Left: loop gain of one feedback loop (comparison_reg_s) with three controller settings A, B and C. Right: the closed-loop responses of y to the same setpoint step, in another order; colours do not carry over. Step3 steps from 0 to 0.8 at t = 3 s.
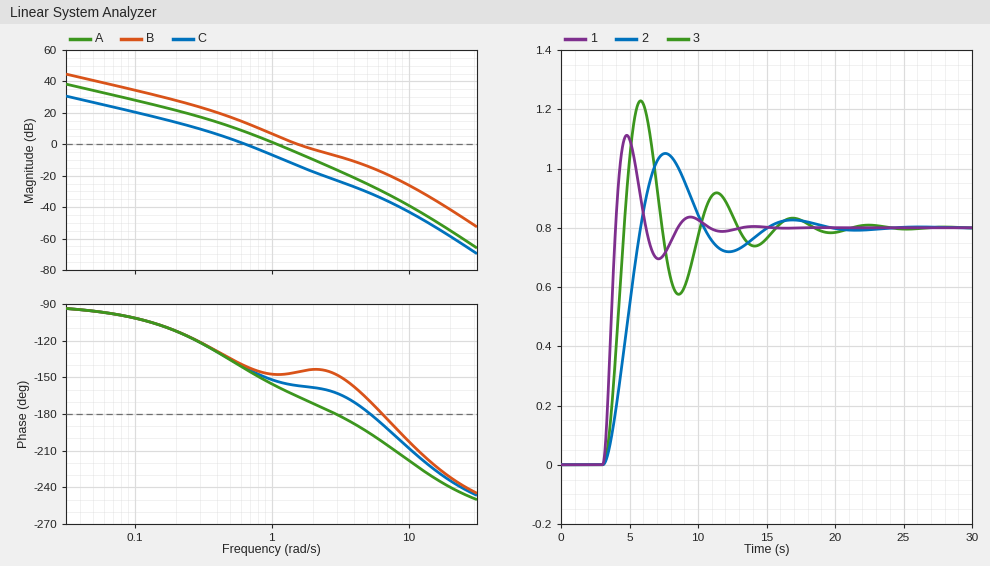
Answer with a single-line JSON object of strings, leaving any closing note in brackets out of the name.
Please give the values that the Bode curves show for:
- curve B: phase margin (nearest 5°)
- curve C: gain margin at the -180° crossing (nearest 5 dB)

{"curve B: phase margin": "35°", "curve C: gain margin at the -180° crossing": "30 dB"}
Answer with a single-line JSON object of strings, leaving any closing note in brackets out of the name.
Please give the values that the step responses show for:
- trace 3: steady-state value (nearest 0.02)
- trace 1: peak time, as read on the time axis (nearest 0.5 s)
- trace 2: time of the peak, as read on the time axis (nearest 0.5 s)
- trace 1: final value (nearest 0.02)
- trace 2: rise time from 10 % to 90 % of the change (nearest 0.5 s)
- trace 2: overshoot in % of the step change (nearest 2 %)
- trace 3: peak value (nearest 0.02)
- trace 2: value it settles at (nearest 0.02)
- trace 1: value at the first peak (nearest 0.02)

{"trace 3: steady-state value": "0.80", "trace 1: peak time, as read on the time axis": "5.0 s", "trace 2: time of the peak, as read on the time axis": "7.5 s", "trace 1: final value": "0.80", "trace 2: rise time from 10 % to 90 % of the change": "2.0 s", "trace 2: overshoot in % of the step change": "32 %", "trace 3: peak value": "1.22", "trace 2: value it settles at": "0.80", "trace 1: value at the first peak": "1.12"}
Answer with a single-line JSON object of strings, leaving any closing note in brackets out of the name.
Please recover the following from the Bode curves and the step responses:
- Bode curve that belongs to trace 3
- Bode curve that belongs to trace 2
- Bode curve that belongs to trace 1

{"Bode curve that belongs to trace 3": "A", "Bode curve that belongs to trace 2": "C", "Bode curve that belongs to trace 1": "B"}
